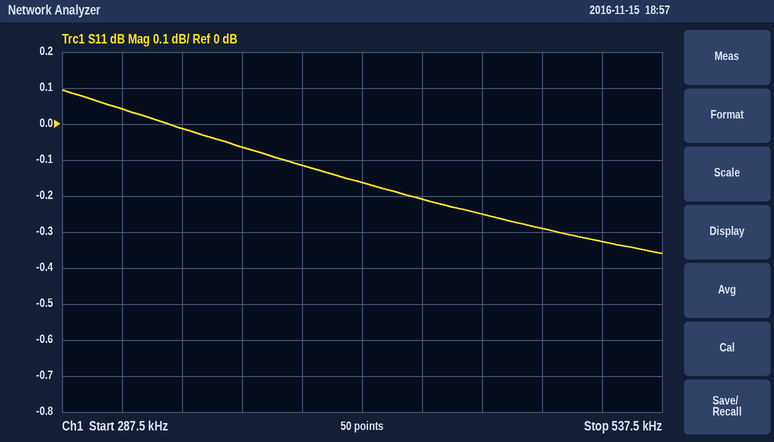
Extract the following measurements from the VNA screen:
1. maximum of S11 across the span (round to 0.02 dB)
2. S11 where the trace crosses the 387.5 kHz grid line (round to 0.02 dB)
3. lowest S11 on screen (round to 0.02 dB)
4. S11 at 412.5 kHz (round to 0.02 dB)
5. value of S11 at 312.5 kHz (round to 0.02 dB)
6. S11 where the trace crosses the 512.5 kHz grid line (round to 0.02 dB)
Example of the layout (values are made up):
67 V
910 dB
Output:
0.10 dB
-0.12 dB
-0.36 dB
-0.16 dB
0.04 dB
-0.32 dB
